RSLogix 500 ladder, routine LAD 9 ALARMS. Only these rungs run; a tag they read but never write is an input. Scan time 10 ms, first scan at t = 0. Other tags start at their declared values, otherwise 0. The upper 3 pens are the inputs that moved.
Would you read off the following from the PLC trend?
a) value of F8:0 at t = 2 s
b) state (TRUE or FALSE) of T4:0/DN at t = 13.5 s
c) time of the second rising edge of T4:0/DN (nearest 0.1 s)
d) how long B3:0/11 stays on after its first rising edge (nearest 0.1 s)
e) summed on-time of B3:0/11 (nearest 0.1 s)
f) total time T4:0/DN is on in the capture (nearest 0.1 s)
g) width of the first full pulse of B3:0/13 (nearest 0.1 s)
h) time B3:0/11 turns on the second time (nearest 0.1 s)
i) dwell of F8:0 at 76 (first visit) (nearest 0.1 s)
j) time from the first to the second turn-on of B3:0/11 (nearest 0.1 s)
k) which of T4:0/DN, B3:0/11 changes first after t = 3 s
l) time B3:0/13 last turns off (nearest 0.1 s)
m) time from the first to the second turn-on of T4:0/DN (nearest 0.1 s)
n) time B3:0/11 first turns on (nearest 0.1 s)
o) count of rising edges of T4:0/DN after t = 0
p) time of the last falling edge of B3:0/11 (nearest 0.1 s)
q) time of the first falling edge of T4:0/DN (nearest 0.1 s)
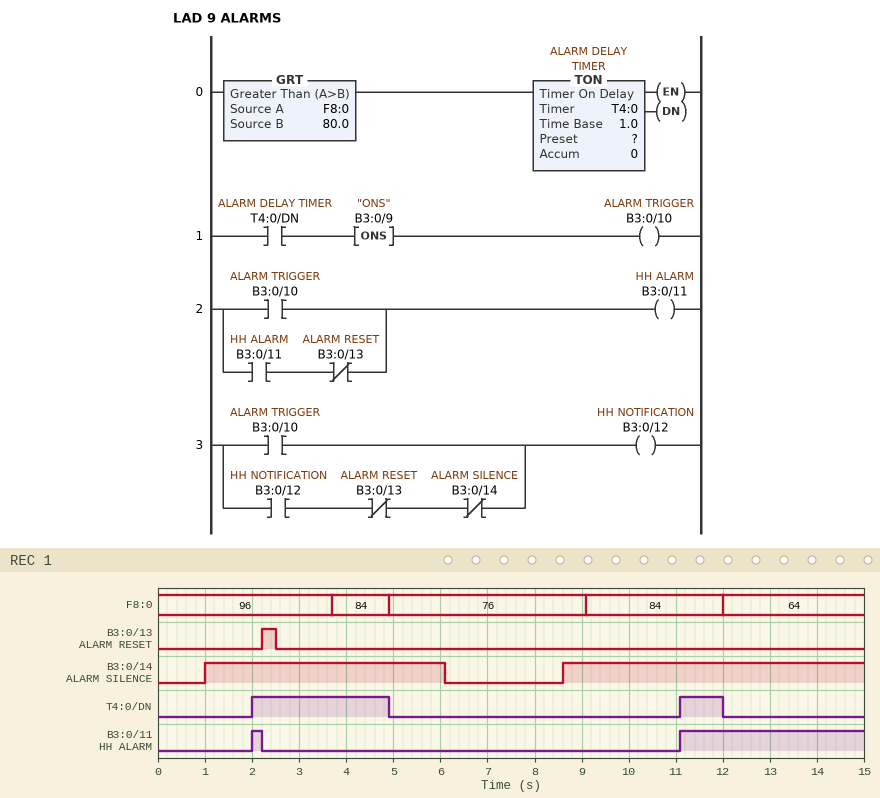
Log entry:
96
FALSE
11.1 s
0.2 s
4.1 s
3.8 s
0.3 s
11.1 s
4.2 s
9.1 s
T4:0/DN
2.5 s
9.1 s
2.0 s
2
2.2 s
4.9 s
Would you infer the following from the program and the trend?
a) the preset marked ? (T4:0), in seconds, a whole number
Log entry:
2 s
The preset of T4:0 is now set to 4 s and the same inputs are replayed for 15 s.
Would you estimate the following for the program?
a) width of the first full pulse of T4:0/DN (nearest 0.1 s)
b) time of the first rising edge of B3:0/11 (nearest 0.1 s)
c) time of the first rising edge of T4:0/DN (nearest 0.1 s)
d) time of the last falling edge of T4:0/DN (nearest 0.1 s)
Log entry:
0.9 s
4.0 s
4.0 s
4.9 s
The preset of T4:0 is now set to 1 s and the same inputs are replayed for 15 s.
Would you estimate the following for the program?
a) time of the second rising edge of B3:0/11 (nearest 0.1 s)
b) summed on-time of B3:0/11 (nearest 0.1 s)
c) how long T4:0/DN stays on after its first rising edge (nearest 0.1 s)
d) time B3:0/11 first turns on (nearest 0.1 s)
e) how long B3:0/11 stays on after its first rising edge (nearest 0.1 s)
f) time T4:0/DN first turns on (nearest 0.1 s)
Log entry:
10.1 s
6.1 s
3.9 s
1.0 s
1.2 s
1.0 s
